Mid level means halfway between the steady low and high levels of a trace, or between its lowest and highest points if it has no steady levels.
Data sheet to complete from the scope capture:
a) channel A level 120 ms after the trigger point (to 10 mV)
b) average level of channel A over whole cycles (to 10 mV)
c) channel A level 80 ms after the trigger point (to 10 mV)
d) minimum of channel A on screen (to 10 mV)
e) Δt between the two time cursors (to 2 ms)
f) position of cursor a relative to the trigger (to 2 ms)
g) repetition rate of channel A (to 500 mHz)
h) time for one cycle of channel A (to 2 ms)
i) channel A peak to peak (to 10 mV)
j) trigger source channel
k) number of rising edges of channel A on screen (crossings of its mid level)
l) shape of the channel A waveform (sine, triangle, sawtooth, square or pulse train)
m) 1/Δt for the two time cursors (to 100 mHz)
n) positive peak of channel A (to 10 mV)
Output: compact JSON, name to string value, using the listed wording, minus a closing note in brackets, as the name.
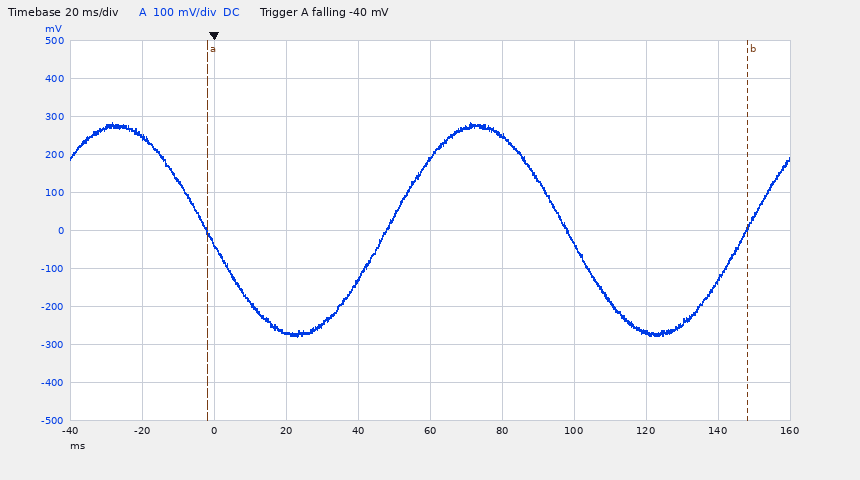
{"channel A level 120 ms after the trigger point": "-270 mV", "average level of channel A over whole cycles": "0 mV", "channel A level 80 ms after the trigger point": "250 mV", "minimum of channel A on screen": "-280 mV", "Δt between the two time cursors": "150 ms", "position of cursor a relative to the trigger": "-2 ms", "repetition rate of channel A": "10.0 Hz", "time for one cycle of channel A": "100 ms", "channel A peak to peak": "560 mV", "trigger source channel": "channel A", "number of rising edges of channel A on screen": "2", "shape of the channel A waveform": "sine", "1/Δt for the two time cursors": "6.7 Hz", "positive peak of channel A": "280 mV"}
